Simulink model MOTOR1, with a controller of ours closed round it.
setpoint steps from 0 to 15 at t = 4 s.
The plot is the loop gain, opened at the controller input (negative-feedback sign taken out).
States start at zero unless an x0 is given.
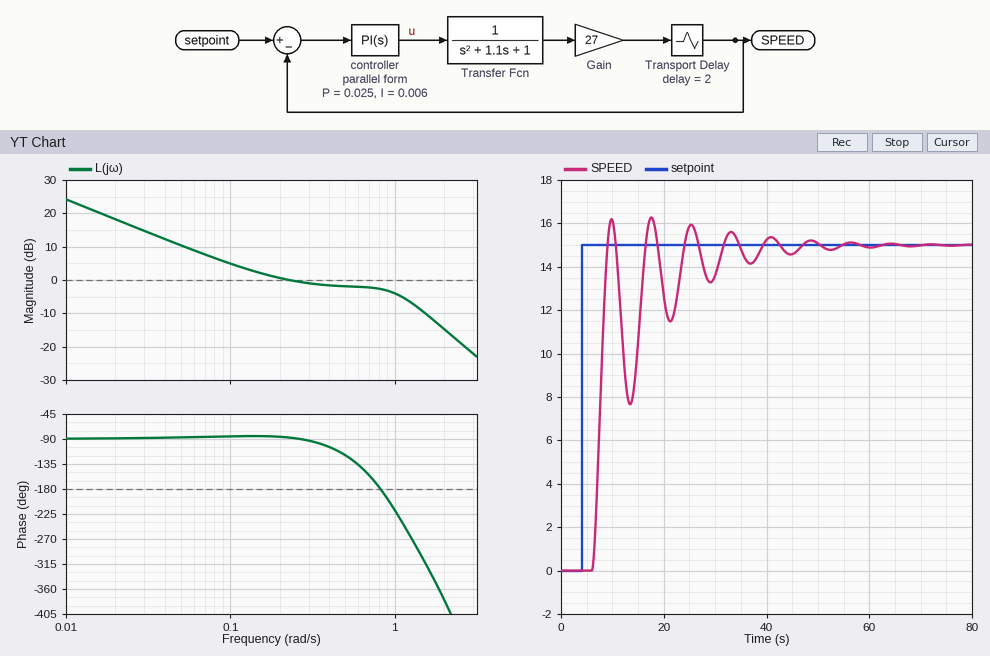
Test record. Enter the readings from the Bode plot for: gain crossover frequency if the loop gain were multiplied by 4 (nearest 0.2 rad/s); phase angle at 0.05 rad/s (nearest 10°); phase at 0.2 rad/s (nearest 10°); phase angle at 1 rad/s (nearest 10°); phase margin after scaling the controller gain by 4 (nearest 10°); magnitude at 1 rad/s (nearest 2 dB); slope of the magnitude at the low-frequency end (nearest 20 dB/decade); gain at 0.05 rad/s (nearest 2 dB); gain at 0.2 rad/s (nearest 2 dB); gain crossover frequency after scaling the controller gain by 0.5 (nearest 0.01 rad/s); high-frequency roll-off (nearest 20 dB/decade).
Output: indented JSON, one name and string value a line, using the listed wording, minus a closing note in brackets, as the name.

{
  "gain crossover frequency if the loop gain were multiplied by 4": "1.8 rad/s",
  "phase angle at 0.05 rad/s": "-90°",
  "phase at 0.2 rad/s": "-90°",
  "phase angle at 1 rad/s": "-220°",
  "phase margin after scaling the controller gain by 4": "-160°",
  "magnitude at 1 rad/s": "-4 dB",
  "slope of the magnitude at the low-frequency end": "-20 dB/decade",
  "gain at 0.05 rad/s": "10 dB",
  "gain at 0.2 rad/s": "0 dB",
  "gain crossover frequency after scaling the controller gain by 0.5": "0.09 rad/s",
  "high-frequency roll-off": "-40 dB/decade"
}
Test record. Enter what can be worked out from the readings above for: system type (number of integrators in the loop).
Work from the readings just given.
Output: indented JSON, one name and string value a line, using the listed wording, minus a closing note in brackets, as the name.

{
  "system type": "1"
}
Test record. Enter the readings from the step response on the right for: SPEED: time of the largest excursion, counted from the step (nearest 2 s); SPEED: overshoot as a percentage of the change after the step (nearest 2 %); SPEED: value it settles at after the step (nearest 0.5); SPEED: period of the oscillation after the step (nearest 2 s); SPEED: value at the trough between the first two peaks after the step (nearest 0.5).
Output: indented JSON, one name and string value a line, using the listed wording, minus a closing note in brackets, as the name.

{
  "SPEED: time of the largest excursion, counted from the step": "14 s",
  "SPEED: overshoot as a percentage of the change after the step": "8 %",
  "SPEED: value it settles at after the step": "15.0",
  "SPEED: period of the oscillation after the step": "8 s",
  "SPEED: value at the trough between the first two peaks after the step": "7.5"
}
